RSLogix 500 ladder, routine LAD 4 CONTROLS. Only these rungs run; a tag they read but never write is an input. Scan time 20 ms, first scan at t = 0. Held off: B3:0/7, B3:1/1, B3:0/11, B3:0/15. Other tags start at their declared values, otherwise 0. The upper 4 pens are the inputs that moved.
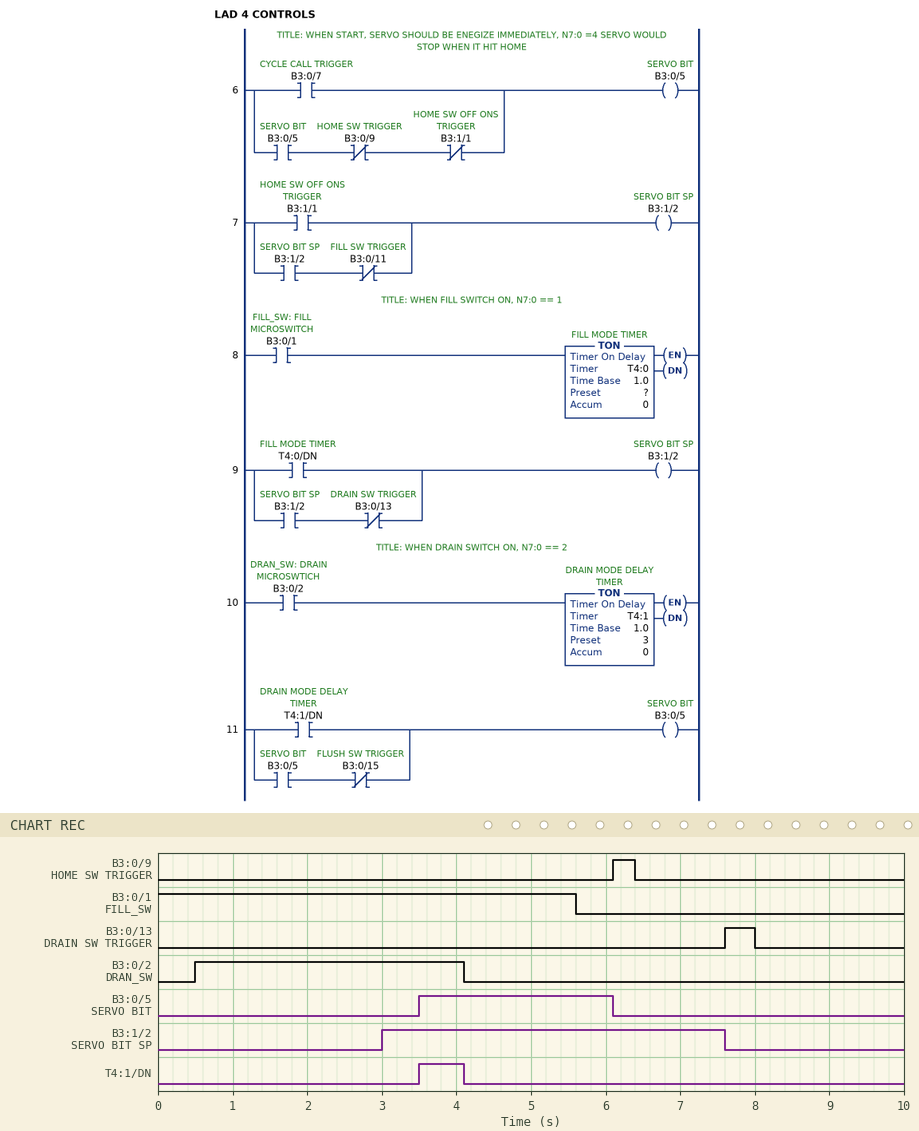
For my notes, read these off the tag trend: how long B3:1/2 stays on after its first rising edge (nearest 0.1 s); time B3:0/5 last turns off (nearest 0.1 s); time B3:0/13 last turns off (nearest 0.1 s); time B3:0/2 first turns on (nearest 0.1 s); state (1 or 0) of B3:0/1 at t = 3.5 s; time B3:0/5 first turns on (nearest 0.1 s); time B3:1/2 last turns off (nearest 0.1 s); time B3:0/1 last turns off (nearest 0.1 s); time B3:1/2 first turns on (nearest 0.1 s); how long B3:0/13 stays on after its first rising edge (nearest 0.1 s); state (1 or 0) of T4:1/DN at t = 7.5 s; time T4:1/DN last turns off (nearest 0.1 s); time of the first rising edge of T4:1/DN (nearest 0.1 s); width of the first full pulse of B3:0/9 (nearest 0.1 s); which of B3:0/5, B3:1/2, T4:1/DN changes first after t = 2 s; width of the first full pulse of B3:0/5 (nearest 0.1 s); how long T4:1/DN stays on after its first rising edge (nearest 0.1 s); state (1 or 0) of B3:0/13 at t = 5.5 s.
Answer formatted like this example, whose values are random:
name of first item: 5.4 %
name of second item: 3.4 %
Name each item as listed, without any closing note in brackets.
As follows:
how long B3:1/2 stays on after its first rising edge: 4.6 s
time B3:0/5 last turns off: 6.1 s
time B3:0/13 last turns off: 8.0 s
time B3:0/2 first turns on: 0.5 s
state (1 or 0) of B3:0/1 at t = 3.5 s: 1
time B3:0/5 first turns on: 3.5 s
time B3:1/2 last turns off: 7.6 s
time B3:0/1 last turns off: 5.6 s
time B3:1/2 first turns on: 3.0 s
how long B3:0/13 stays on after its first rising edge: 0.4 s
state (1 or 0) of T4:1/DN at t = 7.5 s: 0
time T4:1/DN last turns off: 4.1 s
time of the first rising edge of T4:1/DN: 3.5 s
width of the first full pulse of B3:0/9: 0.3 s
which of B3:0/5, B3:1/2, T4:1/DN changes first after t = 2 s: B3:1/2
width of the first full pulse of B3:0/5: 2.6 s
how long T4:1/DN stays on after its first rising edge: 0.6 s
state (1 or 0) of B3:0/13 at t = 5.5 s: 0
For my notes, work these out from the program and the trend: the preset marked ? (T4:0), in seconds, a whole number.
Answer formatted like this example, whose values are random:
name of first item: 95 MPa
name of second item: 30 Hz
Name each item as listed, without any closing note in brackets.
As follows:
the preset marked ? (T4:0), in seconds, a whole number: 3 s
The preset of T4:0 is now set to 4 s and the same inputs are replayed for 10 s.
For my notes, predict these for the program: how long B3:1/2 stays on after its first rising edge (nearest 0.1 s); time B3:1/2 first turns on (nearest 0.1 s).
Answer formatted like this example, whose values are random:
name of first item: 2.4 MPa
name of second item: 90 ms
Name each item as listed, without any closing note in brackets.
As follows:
how long B3:1/2 stays on after its first rising edge: 3.6 s
time B3:1/2 first turns on: 4.0 s
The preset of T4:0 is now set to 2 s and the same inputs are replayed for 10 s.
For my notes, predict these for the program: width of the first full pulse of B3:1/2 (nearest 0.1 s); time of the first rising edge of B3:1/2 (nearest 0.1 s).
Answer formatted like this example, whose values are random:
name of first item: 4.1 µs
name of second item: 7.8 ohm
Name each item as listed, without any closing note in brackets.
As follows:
width of the first full pulse of B3:1/2: 5.6 s
time of the first rising edge of B3:1/2: 2.0 s
